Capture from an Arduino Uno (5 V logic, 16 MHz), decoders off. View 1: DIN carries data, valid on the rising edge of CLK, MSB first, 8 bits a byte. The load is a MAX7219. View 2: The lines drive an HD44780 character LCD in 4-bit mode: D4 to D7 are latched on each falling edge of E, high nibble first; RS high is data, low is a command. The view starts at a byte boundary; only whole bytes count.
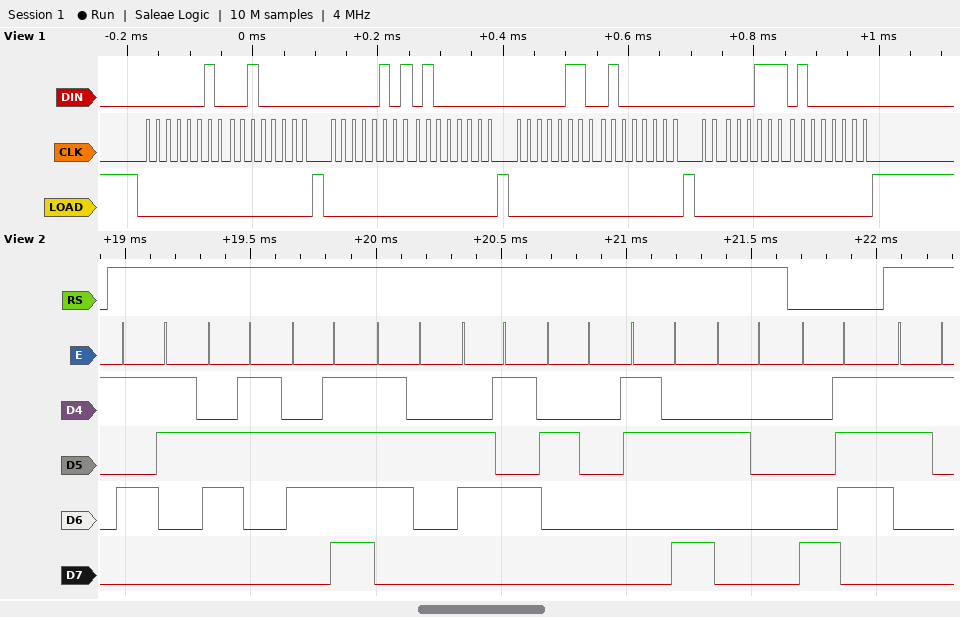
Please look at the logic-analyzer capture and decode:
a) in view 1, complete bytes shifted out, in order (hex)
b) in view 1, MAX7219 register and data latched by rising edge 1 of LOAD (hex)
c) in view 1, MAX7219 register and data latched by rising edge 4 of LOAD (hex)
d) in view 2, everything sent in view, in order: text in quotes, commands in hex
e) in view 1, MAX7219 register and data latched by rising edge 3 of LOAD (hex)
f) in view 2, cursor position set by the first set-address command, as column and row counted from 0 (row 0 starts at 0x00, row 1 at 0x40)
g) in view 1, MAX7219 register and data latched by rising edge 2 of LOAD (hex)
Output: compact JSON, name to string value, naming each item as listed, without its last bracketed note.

{"in view 1, complete bytes shifted out, in order": "02 20 05 40 06 40 07 40", "in view 1, MAX7219 register and data latched by rising edge 1 of LOAD": "register 0x2, data 0x20", "in view 1, MAX7219 register and data latched by rising edge 4 of LOAD": "register 0x7, data 0x40", "in view 2, everything sent in view, in order: text in quotes, commands in hex": "\"Score : \" 0x87 \"1\"", "in view 1, MAX7219 register and data latched by rising edge 3 of LOAD": "register 0x6, data 0x40", "in view 2, cursor position set by the first set-address command, as column and row counted from 0": "column 7, row 0", "in view 1, MAX7219 register and data latched by rising edge 2 of LOAD": "register 0x5, data 0x40"}
